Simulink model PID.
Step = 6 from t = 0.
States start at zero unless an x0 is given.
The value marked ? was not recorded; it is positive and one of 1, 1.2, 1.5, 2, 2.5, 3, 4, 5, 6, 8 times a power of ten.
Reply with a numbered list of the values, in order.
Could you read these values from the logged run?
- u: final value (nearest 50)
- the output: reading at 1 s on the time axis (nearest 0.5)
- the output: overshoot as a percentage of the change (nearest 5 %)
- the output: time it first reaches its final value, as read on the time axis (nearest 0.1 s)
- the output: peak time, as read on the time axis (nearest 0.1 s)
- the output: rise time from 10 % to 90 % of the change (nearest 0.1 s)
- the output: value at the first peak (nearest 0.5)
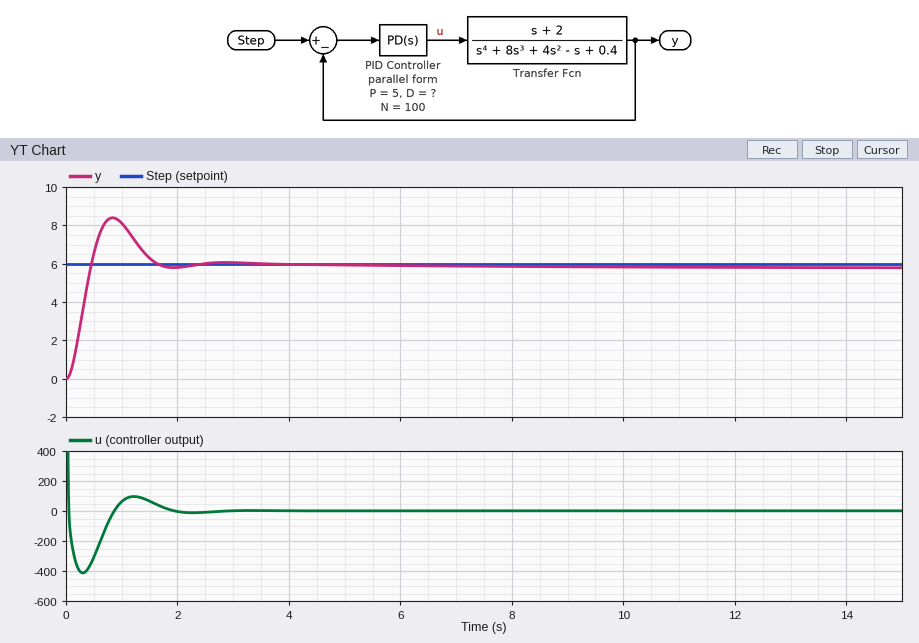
1. 0
2. 8.0
3. 45 %
4. 0.4 s
5. 0.8 s
6. 0.3 s
7. 8.5
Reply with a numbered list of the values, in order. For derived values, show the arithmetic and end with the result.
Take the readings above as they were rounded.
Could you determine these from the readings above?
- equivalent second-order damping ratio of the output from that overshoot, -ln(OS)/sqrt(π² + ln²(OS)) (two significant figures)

1. ln(0.45) = -0.799; 0.799 / sqrt(9.870 + 0.638) = 0.25
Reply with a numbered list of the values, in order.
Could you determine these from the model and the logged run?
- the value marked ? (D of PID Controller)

1. 25
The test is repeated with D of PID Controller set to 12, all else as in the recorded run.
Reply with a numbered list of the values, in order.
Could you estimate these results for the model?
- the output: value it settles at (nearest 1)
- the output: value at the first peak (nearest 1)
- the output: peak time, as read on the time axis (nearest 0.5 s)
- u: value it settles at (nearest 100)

1. 6
2. 9
3. 1.5 s
4. 0
